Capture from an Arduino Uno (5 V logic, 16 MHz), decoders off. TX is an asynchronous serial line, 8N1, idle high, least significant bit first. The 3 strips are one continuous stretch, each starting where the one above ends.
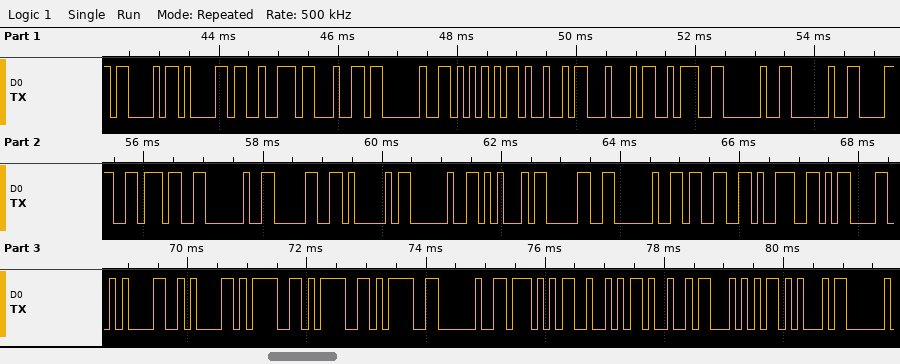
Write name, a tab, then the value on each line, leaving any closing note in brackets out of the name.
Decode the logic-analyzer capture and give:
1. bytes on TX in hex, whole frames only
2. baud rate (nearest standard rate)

bytes on TX in hex, whole frames only	43 61 72 64 20 55 49 44 3A 20 20 38 37 20 30 41 20 45 30 20 33 39 0D 0A 0A 3D 3D 3D 20 57 52 49 54 45
baud rate	9600 baud
